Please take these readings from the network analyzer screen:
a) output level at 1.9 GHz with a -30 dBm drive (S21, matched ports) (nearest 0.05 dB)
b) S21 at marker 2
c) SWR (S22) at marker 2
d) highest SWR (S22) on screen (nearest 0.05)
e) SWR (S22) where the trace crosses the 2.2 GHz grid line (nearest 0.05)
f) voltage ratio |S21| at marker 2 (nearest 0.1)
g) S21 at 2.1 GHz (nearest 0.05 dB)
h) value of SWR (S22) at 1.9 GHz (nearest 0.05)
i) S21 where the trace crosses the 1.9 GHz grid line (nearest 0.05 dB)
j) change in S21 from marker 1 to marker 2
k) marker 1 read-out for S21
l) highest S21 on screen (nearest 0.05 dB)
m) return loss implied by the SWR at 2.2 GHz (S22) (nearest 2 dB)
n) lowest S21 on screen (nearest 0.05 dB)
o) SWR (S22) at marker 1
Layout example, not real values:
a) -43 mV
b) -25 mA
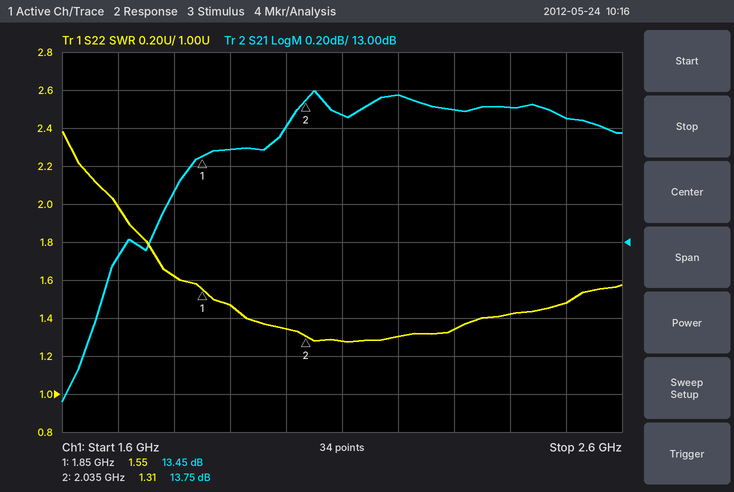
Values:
a) -16.50 dBm
b) 13.75 dB
c) 1.31
d) 2.40
e) 1.30
f) 4.9
g) 13.65 dB
h) 1.45
i) 13.50 dB
j) 0.30 dB
k) 13.45 dB
l) 13.80 dB
m) 18 dB
n) 12.15 dB
o) 1.55
